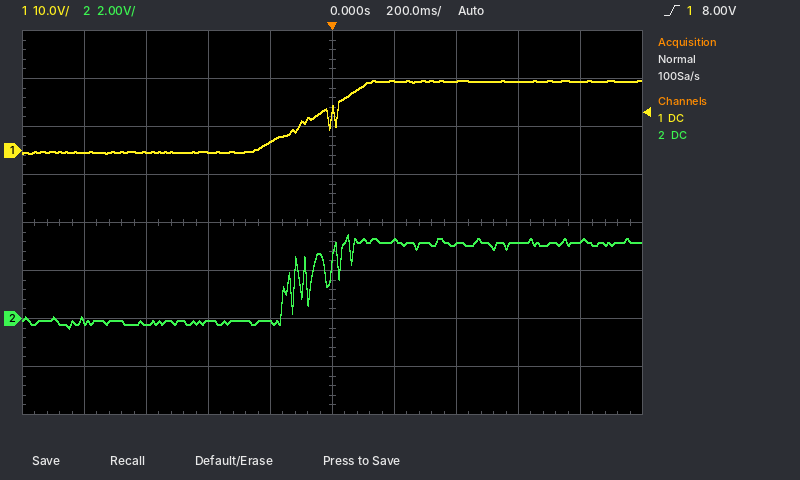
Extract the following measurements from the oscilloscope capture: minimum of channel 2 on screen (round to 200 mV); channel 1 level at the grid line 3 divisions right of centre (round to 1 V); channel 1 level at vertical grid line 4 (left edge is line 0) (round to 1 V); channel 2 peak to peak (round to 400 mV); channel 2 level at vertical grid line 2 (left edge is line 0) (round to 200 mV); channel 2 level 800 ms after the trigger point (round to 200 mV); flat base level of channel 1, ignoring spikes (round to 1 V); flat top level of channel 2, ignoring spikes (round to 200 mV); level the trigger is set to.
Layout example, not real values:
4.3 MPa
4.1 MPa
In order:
-400 mV
14 V
2 V
4.0 V
-200 mV
3.2 V
0 V
3.2 V
8.00 V
